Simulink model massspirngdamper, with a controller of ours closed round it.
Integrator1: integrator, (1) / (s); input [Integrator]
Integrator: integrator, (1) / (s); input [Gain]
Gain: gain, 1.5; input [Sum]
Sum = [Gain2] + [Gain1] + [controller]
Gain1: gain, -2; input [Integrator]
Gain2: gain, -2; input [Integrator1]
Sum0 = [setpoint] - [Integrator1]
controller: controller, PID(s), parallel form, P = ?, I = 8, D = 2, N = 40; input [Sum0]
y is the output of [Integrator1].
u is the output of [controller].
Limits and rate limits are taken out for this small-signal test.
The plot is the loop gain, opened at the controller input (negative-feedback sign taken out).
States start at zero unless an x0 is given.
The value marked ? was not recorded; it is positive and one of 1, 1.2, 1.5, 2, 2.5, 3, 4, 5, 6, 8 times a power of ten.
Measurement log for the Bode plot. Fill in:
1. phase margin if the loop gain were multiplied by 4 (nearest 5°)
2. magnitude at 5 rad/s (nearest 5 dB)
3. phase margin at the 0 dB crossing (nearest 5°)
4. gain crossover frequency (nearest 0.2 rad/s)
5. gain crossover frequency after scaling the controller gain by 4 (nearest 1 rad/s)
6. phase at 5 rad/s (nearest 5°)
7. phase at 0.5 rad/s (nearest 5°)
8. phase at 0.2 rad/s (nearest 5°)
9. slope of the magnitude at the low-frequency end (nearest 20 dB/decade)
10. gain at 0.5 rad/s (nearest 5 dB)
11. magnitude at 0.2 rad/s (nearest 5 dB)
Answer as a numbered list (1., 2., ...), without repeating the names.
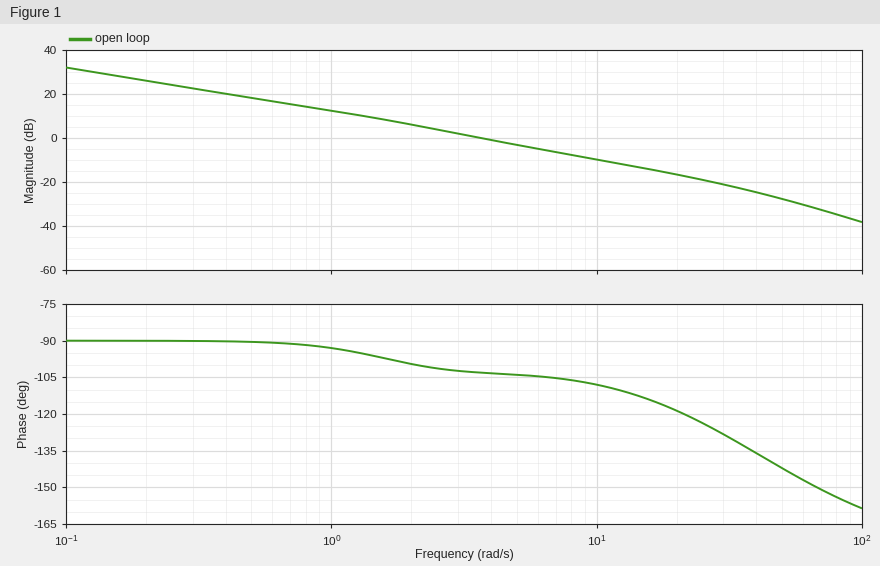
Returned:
1. 70°
2. -5 dB
3. 75°
4. 3.6 rad/s
5. 13 rad/s
6. -105°
7. -90°
8. -90°
9. -20 dB/decade
10. 20 dB
11. 25 dB
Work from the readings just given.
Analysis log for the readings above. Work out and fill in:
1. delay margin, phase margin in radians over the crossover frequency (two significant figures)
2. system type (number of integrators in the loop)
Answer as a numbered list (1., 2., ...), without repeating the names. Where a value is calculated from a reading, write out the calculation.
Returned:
1. 75 × π / 180 / 3.6 = 0.36 s
2. 1
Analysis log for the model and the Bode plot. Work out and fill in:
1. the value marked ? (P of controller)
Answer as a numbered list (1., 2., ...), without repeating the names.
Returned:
1. 8
